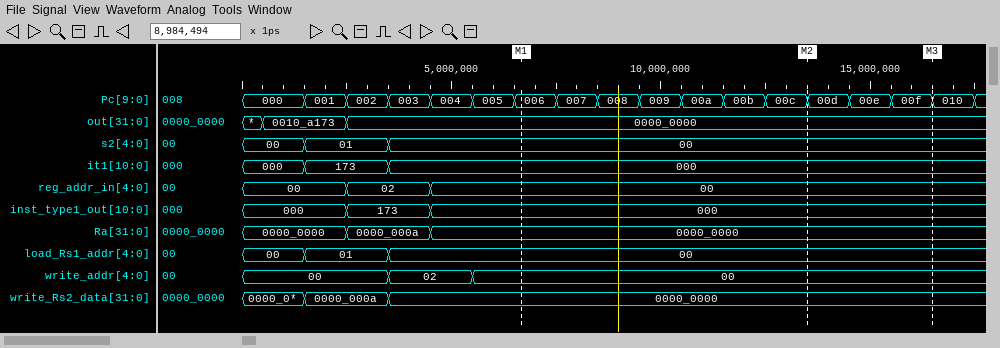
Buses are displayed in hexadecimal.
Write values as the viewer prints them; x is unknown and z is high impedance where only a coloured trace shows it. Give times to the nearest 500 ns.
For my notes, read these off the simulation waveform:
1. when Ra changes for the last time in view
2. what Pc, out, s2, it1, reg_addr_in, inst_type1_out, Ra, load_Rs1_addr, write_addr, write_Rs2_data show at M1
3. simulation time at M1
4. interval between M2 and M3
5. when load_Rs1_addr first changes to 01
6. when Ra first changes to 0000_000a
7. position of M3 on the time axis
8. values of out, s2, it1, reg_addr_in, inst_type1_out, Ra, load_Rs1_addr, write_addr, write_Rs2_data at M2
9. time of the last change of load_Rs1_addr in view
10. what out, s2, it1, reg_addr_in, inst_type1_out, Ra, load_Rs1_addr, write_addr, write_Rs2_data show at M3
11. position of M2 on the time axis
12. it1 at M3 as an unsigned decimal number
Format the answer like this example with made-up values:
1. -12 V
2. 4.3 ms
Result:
1. 4500 ns
2. Pc=006, out=0000_0000, s2=00, it1=000, reg_addr_in=00, inst_type1_out=000, Ra=0000_0000, load_Rs1_addr=00, write_addr=00, write_Rs2_data=0000_0000
3. 6500 ns
4. 3000 ns
5. 1500 ns
6. 2500 ns
7. 16500 ns
8. out=0000_0000, s2=00, it1=000, reg_addr_in=00, inst_type1_out=000, Ra=0000_0000, load_Rs1_addr=00, write_addr=00, write_Rs2_data=0000_0000
9. 3500 ns
10. out=0000_0000, s2=00, it1=000, reg_addr_in=00, inst_type1_out=000, Ra=0000_0000, load_Rs1_addr=00, write_addr=00, write_Rs2_data=0000_0000
11. 13500 ns
12. 0
